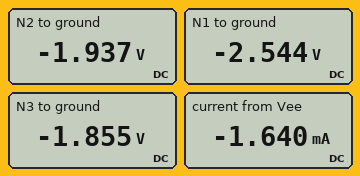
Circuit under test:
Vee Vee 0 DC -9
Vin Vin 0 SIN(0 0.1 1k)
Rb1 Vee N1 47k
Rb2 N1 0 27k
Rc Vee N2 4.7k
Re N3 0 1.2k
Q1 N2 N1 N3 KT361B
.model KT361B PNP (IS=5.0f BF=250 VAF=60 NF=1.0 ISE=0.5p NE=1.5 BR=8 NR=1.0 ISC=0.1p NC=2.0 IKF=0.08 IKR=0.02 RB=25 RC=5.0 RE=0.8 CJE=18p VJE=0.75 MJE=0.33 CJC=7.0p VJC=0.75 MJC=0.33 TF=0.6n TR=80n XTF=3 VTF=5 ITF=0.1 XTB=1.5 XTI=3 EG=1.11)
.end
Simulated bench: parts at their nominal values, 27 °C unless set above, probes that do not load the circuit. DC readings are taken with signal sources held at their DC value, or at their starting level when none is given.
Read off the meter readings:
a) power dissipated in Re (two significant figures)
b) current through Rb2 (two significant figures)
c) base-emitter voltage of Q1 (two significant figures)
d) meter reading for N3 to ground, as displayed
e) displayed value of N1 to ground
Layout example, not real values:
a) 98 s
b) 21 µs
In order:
a) 2.9 mW
b) 94 µA
c) -690 mV
d) -1.855 V
e) -2.544 V
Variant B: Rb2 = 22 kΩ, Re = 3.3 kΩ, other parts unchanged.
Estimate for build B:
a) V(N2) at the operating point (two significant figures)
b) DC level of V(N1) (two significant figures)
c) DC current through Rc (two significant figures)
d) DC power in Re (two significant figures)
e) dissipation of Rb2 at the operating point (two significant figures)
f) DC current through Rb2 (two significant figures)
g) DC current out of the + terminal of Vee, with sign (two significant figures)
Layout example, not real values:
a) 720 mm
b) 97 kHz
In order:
a) -6.2 V
b) -2.7 V
c) 590 µA
d) 1.2 mW
e) 320 µW
f) 120 µA
g) -730 µA
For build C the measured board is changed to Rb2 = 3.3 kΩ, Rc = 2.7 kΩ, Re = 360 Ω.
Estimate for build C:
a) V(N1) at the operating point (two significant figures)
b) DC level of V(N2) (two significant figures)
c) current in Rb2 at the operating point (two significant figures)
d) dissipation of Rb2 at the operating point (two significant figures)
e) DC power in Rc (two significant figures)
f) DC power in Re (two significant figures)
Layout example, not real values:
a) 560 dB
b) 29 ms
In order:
a) -590 mV
b) -8.9 V
c) 180 µA
d) 100 µW
e) 1.9 µW
f) 280 nW
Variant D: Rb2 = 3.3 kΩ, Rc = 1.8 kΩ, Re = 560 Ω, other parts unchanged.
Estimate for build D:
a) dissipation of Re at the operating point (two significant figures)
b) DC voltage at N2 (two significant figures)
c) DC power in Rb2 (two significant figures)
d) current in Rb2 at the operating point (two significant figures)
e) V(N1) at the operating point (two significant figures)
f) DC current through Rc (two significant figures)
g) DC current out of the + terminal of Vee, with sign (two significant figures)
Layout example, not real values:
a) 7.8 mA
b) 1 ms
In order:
a) 340 nW
b) -9.0 V
c) 100 µW
d) 180 µA
e) -590 mV
f) 23 µA
g) -200 µA
